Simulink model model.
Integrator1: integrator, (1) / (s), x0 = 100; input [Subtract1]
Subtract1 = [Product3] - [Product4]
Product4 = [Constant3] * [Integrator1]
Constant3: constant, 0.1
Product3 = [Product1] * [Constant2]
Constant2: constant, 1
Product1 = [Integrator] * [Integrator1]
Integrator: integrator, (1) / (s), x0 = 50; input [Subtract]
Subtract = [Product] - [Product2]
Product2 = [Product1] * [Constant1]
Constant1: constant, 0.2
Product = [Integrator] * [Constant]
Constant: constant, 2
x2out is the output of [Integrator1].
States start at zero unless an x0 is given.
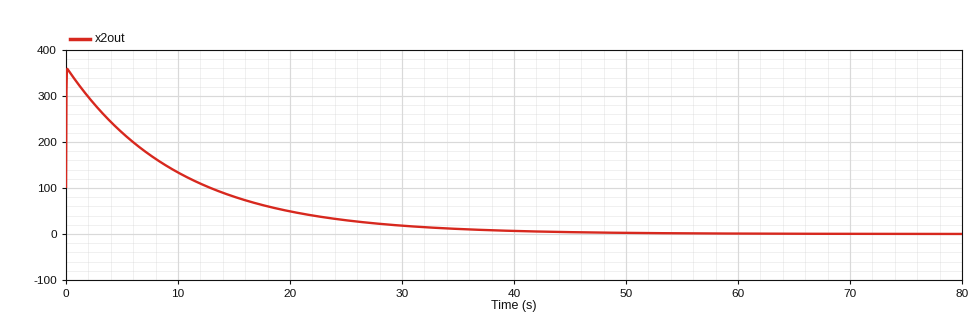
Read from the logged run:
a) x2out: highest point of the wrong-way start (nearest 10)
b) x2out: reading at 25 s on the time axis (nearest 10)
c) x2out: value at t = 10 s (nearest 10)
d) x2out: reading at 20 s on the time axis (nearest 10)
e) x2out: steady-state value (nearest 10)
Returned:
360
30
130
50
0
